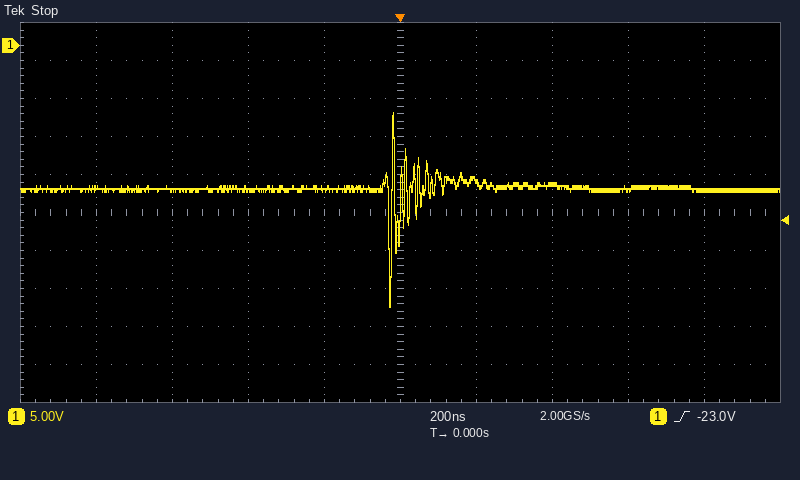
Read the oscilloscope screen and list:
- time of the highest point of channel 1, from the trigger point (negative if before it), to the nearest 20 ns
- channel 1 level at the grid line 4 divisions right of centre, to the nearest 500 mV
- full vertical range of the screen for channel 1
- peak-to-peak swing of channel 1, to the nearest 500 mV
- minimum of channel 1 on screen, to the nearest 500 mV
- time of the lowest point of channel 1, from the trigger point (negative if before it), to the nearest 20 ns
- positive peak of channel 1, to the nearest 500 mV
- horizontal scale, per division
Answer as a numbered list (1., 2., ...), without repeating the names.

1. -20 ns
2. -19.0 V
3. 50 V
4. 25.5 V
5. -34.5 V
6. -20 ns
7. -9.0 V
8. 200 ns
